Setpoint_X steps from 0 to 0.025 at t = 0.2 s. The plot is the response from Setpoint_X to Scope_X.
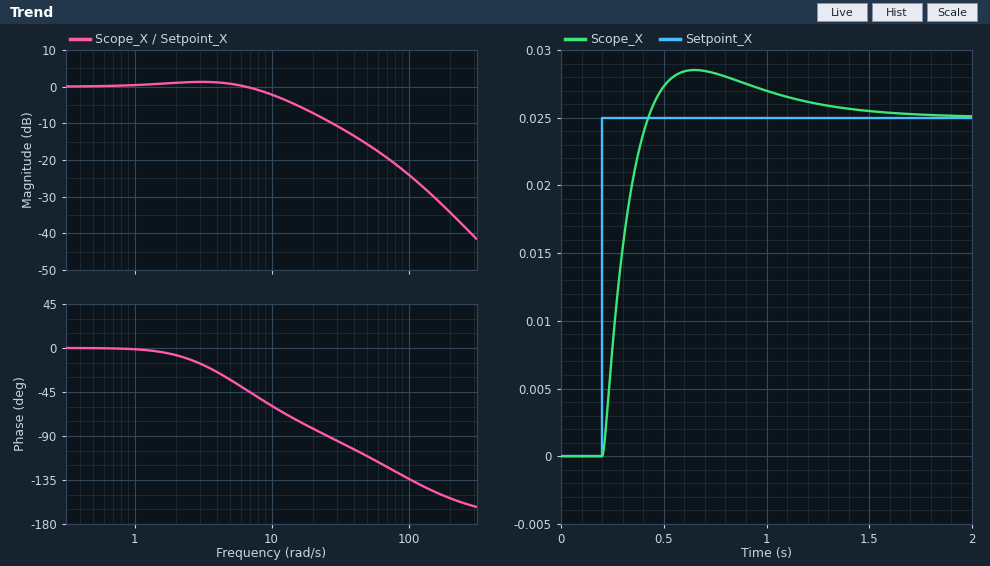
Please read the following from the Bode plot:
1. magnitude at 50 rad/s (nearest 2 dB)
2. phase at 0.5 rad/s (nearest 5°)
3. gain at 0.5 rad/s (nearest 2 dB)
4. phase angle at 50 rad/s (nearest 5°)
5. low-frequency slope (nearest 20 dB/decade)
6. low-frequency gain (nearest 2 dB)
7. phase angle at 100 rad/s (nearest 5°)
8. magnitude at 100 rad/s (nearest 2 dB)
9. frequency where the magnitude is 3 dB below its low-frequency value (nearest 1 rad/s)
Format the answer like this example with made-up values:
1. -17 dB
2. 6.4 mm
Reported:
1. -16 dB
2. 0°
3. 0 dB
4. -110°
5. 0 dB/decade
6. 0 dB
7. -135°
8. -24 dB
9. 11 rad/s
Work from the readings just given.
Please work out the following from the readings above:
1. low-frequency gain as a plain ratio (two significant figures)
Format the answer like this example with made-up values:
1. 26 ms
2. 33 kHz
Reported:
1. 1.0
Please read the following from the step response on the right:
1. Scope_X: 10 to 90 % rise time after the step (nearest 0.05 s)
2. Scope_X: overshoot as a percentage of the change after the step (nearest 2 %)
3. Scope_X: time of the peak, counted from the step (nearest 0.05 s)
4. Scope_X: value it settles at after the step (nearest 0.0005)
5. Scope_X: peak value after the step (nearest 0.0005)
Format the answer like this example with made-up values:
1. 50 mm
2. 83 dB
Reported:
1. 0.15 s
2. 14 %
3. 0.45 s
4. 0.0250
5. 0.0285
